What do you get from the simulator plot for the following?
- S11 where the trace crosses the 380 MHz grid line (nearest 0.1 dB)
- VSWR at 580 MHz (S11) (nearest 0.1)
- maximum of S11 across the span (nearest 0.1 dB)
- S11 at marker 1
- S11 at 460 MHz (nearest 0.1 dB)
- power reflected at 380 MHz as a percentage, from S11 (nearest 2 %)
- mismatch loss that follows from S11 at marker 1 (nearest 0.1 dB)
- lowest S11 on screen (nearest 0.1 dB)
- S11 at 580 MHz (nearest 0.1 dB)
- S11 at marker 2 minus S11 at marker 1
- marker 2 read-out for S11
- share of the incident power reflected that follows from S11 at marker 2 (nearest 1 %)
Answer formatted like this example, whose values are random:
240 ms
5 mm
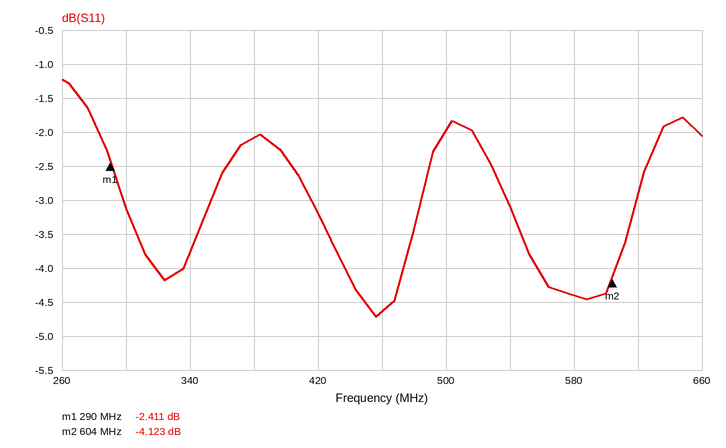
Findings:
-2.1 dB
4.0
-1.2 dB
-2.411 dB
-4.6 dB
62 %
3.7 dB
-4.7 dB
-4.4 dB
-1.712 dB
-4.123 dB
39 %
